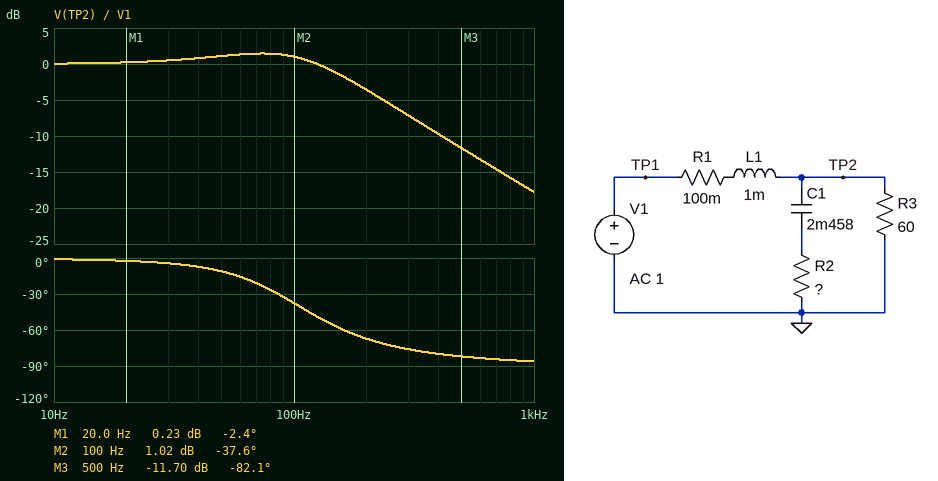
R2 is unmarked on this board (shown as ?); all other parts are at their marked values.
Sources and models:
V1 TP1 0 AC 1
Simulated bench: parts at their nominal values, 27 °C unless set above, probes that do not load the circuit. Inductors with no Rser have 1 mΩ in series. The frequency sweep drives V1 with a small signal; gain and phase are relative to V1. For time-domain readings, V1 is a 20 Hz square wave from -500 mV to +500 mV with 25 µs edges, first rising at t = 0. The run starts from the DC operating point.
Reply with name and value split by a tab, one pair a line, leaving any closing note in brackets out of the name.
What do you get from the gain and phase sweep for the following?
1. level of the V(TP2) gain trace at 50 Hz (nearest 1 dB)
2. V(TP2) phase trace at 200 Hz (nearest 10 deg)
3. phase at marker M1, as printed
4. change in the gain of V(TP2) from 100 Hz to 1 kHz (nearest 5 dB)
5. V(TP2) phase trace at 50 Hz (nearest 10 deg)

level of the V(TP2) gain trace at 50 Hz	1 dB
V(TP2) phase trace at 200 Hz	-70 deg
phase at marker M1, as printed	-2.4 deg
change in the gain of V(TP2) from 100 Hz to 1 kHz	-20 dB
V(TP2) phase trace at 50 Hz	-10 deg
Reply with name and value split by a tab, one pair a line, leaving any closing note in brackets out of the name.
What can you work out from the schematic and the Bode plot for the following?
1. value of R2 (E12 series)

value of R2	0.82 Ω
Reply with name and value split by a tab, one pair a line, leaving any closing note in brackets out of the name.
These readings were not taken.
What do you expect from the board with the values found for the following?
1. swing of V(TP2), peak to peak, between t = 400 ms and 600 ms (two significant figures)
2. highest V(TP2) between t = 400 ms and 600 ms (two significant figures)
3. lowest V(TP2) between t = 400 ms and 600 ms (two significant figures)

swing of V(TP2), peak to peak, between t = 400 ms and 600 ms	1.3 V
highest V(TP2) between t = 400 ms and 600 ms	660 mV
lowest V(TP2) between t = 400 ms and 600 ms	-660 mV
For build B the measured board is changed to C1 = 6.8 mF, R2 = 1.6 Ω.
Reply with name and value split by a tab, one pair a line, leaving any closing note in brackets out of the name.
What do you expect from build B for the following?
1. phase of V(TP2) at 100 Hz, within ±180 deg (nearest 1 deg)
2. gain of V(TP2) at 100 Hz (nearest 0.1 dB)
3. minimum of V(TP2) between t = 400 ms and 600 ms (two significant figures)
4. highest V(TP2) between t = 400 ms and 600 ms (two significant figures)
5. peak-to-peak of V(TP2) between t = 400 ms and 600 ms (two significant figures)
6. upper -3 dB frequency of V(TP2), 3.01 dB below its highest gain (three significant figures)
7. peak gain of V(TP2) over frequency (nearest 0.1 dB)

phase of V(TP2) at 100 Hz, within ±180 deg	-22 deg
gain of V(TP2) at 100 Hz	-0.7 dB
minimum of V(TP2) between t = 400 ms and 600 ms	-500 mV
highest V(TP2) between t = 400 ms and 600 ms	500 mV
peak-to-peak of V(TP2) between t = 400 ms and 600 ms	1.0 V
upper -3 dB frequency of V(TP2), 3.01 dB below its highest gain	247 Hz
peak gain of V(TP2) over frequency	0 dB
